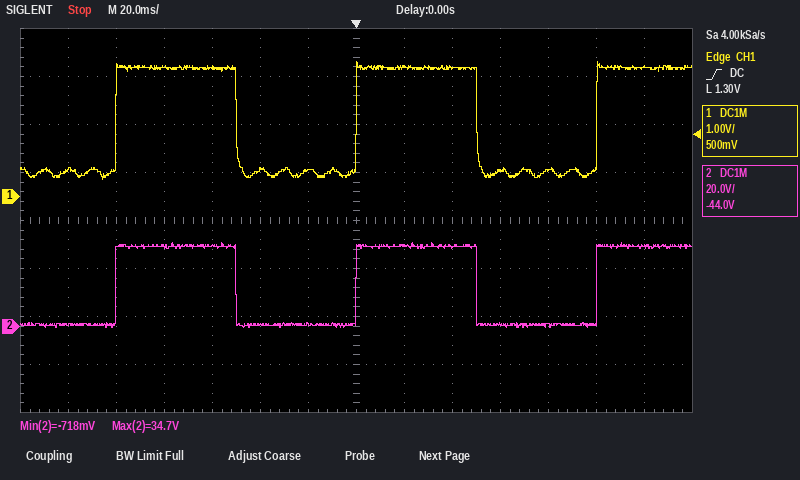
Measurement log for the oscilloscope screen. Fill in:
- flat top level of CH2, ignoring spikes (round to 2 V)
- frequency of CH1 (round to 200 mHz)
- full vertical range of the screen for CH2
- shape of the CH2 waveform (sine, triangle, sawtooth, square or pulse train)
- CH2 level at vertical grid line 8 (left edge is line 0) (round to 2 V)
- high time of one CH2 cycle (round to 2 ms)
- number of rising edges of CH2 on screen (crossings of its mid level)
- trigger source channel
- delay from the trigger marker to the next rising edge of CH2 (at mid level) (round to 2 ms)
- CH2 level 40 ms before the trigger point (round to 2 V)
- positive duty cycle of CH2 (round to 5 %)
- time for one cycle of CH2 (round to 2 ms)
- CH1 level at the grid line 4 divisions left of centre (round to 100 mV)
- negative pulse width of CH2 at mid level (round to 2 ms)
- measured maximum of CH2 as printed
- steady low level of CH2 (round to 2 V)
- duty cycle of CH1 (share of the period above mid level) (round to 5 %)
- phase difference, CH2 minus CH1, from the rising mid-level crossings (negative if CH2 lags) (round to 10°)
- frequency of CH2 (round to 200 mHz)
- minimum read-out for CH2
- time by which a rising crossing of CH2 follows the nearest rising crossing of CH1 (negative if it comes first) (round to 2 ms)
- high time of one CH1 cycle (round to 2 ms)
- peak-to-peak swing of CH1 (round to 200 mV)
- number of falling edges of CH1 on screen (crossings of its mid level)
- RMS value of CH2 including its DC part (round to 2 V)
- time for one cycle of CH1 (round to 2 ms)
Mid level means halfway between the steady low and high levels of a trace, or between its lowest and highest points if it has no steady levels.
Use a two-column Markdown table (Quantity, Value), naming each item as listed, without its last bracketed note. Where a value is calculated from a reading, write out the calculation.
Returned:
| Quantity | Value |
|---|---|
| flat top level of CH2, ignoring spikes | 34 V |
| frequency of CH1 | 1 / 100 ms ≈ 10.0 Hz |
| full vertical range of the screen for CH2 | 160 V |
| shape of the CH2 waveform | square |
| CH2 level at vertical grid line 8 (left edge is line 0) | 34 V |
| high time of one CH2 cycle | 50 ms |
| number of rising edges of CH2 on screen | 3 |
| trigger source channel | CH1 |
| delay from the trigger marker to the next rising edge of CH2 (at mid level) | 100 ms |
| CH2 level 40 ms before the trigger point | 0 V |
| positive duty cycle of CH2 | 50 ms / 100 ms ≈ 50 % |
| time for one cycle of CH2 | 100 ms |
| CH1 level at the grid line 4 divisions left of centre | 2.7 V |
| negative pulse width of CH2 at mid level | 50 ms |
| measured maximum of CH2 as printed | 34.7 V |
| steady low level of CH2 | 0 V |
| duty cycle of CH1 (share of the period above mid level) | 50 ms / 100 ms ≈ 50 % |
| phase difference, CH2 minus CH1, from the rising mid-level crossings (negative if CH2 lags) | −360° × (0 ms) / 100 ms ≈ 0° |
| frequency of CH2 | 1 / 100 ms ≈ 10.0 Hz |
| minimum read-out for CH2 | -718 mV |
| time by which a rising crossing of CH2 follows the nearest rising crossing of CH1 (negative if it comes first) | 0 ms |
| high time of one CH1 cycle | 50 ms |
| peak-to-peak swing of CH1 | 2.4 V |
| number of falling edges of CH1 on screen | 2 |
| RMS value of CH2 including its DC part | √(0.5 × (34 V)² + 0.5 × (0 V)²) ≈ 24 V |
| time for one cycle of CH1 | 100 ms |
